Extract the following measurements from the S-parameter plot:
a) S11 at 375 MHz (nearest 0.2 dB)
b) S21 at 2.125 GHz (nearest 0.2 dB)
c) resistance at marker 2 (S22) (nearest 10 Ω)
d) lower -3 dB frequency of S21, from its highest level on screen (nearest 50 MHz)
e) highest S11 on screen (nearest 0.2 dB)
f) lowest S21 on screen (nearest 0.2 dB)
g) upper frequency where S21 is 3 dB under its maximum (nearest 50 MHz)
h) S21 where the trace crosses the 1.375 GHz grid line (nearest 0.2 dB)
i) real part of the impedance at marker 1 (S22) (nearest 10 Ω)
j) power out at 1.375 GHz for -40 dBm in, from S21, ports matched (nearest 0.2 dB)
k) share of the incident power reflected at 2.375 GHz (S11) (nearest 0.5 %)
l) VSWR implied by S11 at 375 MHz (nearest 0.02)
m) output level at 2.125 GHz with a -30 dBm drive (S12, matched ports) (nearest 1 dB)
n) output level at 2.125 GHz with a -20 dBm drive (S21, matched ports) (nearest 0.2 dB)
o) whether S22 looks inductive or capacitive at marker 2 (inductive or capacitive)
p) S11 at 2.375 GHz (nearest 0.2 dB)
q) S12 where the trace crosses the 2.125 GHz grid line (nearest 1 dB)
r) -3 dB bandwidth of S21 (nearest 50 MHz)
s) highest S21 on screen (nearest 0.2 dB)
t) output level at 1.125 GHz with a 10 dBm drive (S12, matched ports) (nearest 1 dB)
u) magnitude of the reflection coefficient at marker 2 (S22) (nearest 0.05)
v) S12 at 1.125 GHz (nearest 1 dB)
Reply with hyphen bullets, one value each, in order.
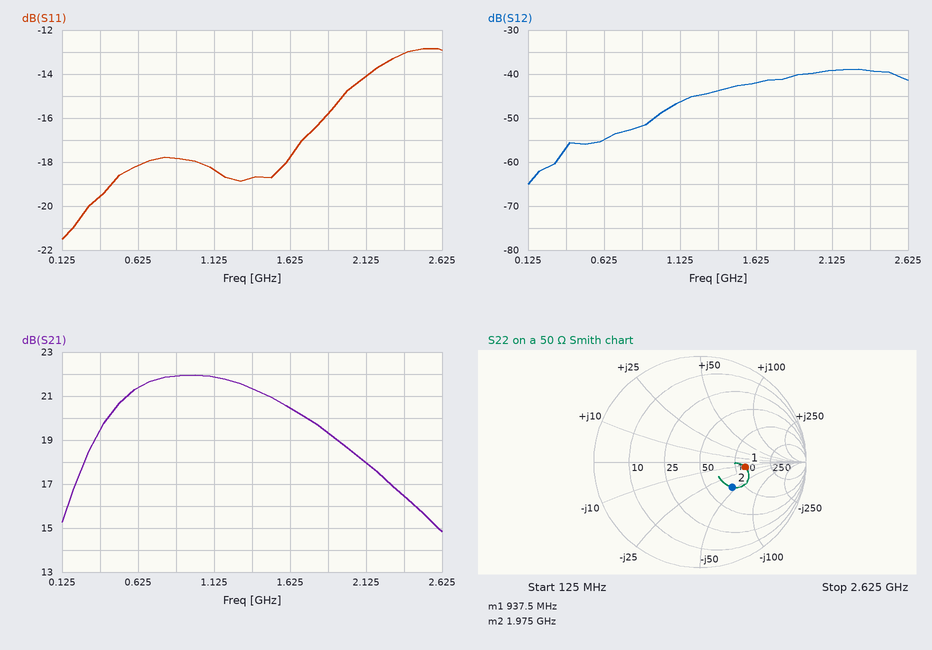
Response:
- -19.6 dB
- 18.0 dB
- 80 Ω
- 350 MHz
- -12.8 dB
- 14.8 dB
- 1.95 GHz
- 21.4 dB
- 120 Ω
- -18.6 dBm
- 5.0 %
- 1.24
- -69 dBm
- -2.0 dBm
- capacitive
- -13.0 dB
- -39 dB
- 1.60 GHz
- 22.0 dB
- -36 dBm
- 0.40
- -46 dB
